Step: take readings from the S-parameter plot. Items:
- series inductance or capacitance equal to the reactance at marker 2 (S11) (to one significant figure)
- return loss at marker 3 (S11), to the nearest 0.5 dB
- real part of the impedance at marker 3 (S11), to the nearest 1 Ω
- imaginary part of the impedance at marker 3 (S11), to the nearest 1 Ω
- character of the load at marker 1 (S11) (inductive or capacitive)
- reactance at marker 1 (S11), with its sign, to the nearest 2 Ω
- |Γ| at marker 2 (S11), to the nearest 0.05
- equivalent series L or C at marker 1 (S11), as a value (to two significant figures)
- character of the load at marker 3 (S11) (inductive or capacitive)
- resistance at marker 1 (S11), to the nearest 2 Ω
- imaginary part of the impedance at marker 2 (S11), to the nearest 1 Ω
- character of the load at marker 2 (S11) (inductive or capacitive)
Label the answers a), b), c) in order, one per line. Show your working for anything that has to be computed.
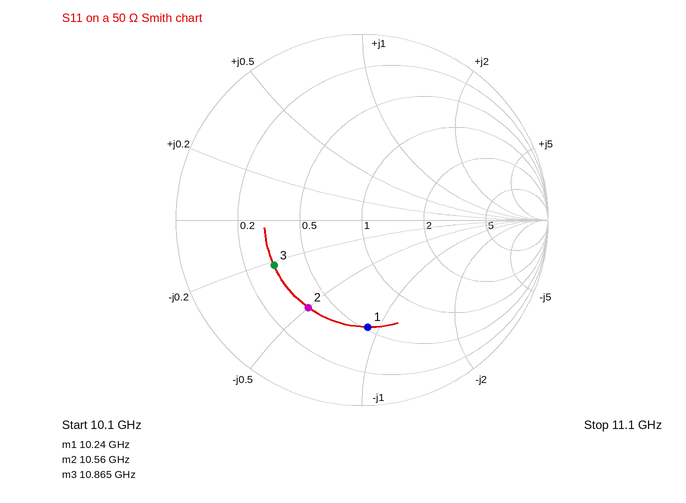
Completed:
a) C = 1/(2π × 10.56 GHz × 25 Ω) ≈ 603 fF, so 600 fF to one significant figure
b) 5.5 dB
c) 16 Ω
d) -11 Ω
e) capacitive
f) -46 Ω
g) 0.55
h) C = 1/(2π × 10.24 GHz × 46 Ω) ≈ 338 fF, so 340 fF to two significant figures
i) capacitive
j) 26 Ω
k) -25 Ω
l) capacitive
